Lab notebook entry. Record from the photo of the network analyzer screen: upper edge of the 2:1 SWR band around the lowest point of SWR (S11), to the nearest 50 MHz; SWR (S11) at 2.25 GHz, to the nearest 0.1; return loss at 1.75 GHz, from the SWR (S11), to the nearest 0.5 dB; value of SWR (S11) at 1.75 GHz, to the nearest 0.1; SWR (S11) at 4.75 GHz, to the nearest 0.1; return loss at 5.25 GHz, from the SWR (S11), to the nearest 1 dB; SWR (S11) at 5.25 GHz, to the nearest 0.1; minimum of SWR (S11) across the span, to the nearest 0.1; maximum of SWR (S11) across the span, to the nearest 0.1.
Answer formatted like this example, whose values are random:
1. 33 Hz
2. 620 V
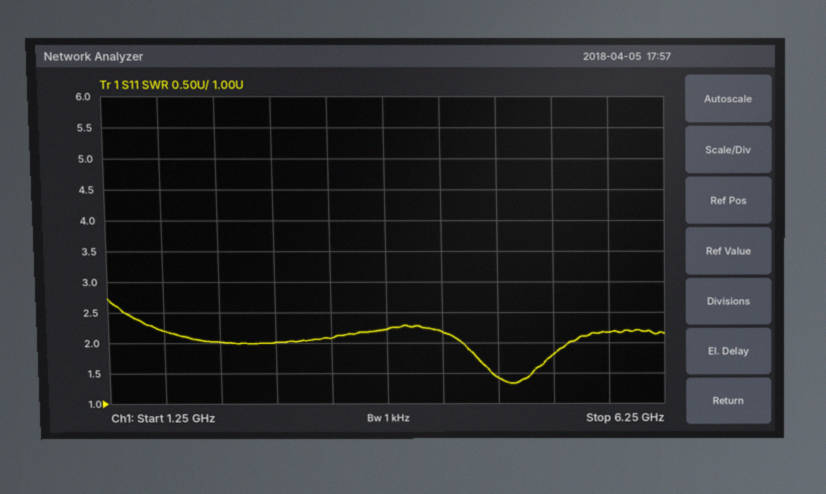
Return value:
1. 5.40 GHz
2. 2.0
3. 8.5 dB
4. 2.2
5. 1.4
6. 11 dB
7. 1.8
8. 1.3
9. 2.7
